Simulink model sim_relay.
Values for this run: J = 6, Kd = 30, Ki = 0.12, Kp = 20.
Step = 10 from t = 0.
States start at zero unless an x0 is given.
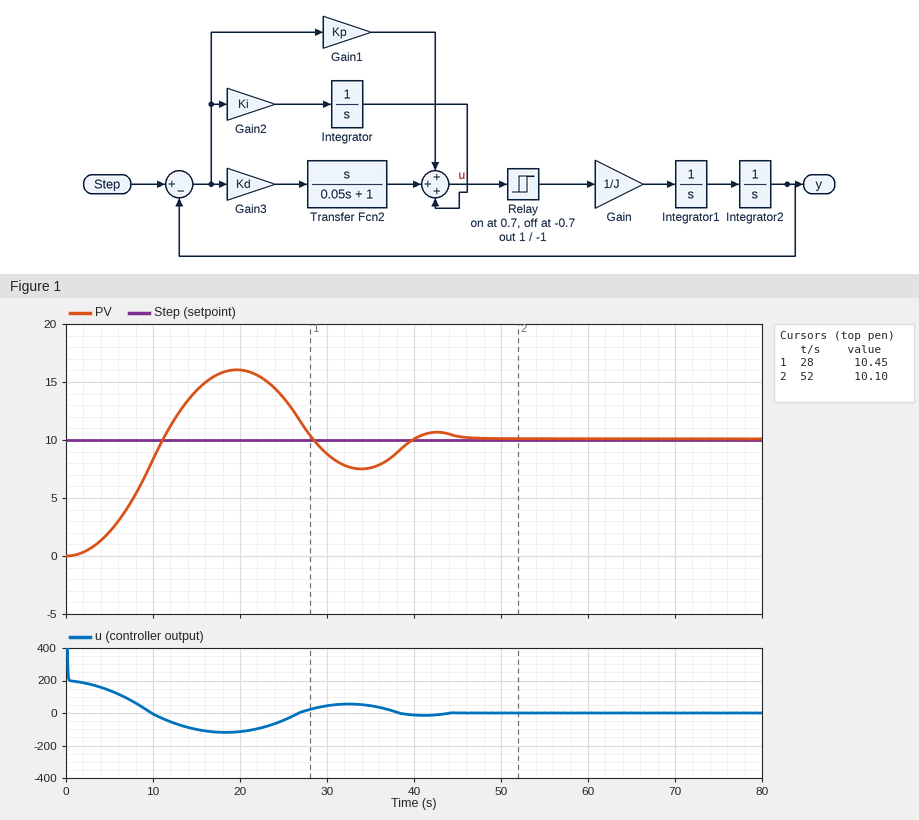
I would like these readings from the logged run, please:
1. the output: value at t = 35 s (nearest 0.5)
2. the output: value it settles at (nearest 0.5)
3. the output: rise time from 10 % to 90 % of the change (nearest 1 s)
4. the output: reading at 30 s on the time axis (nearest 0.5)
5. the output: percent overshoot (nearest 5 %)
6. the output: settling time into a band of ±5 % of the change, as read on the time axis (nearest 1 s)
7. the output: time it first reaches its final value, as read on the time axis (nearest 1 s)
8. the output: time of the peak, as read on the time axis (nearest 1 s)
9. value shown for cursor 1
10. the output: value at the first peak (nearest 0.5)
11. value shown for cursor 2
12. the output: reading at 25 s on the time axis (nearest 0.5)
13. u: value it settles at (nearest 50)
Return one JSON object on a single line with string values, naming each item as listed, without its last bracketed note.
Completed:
{"the output: value at t = 35 s": "7.5", "the output: value it settles at": "10.0", "the output: rise time from 10 % to 90 % of the change": "7 s", "the output: reading at 30 s on the time axis": "9.0", "the output: percent overshoot": "60 %", "the output: settling time into a band of ±5 % of the change, as read on the time axis": "44 s", "the output: time it first reaches its final value, as read on the time axis": "11 s", "the output: time of the peak, as read on the time axis": "20 s", "value shown for cursor 1": "10.45", "the output: value at the first peak": "16.0", "value shown for cursor 2": "10.10", "the output: reading at 25 s on the time axis": "13.5", "u: value it settles at": "0"}
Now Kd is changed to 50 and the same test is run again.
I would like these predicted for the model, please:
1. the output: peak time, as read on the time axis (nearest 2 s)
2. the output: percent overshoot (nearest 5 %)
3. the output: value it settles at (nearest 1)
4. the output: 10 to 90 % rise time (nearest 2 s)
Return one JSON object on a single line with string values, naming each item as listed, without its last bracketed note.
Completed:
{"the output: peak time, as read on the time axis": "18 s", "the output: percent overshoot": "35 %", "the output: value it settles at": "10", "the output: 10 to 90 % rise time": "8 s"}
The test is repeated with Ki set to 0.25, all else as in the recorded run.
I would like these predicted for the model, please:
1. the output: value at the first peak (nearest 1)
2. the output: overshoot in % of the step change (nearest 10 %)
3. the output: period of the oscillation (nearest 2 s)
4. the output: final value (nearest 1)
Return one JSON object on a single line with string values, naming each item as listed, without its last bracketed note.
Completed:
{"the output: value at the first peak": "17", "the output: overshoot in % of the step change": "70 %", "the output: period of the oscillation": "26 s", "the output: final value": "10"}
